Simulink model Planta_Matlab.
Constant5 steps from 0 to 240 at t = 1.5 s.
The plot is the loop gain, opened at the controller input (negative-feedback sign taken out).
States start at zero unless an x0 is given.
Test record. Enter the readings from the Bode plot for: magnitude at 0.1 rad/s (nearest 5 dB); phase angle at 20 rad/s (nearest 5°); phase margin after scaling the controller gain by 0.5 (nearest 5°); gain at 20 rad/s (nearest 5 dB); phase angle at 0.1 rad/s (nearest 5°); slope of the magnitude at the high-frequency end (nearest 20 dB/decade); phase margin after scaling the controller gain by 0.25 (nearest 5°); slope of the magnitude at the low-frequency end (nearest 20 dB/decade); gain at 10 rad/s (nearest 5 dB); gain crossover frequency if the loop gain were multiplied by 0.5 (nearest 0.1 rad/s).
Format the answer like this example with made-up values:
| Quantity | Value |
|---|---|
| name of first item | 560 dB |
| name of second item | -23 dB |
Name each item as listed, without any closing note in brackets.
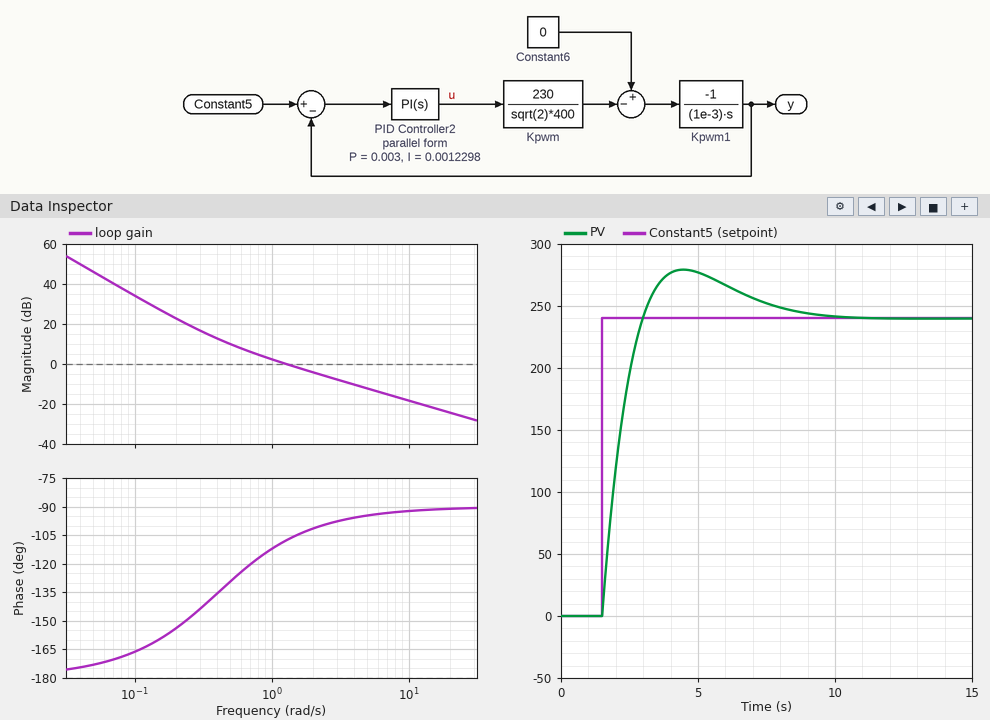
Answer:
| Quantity | Value |
|---|---|
| magnitude at 0.1 rad/s | 35 dB |
| phase angle at 20 rad/s | -90° |
| phase margin after scaling the controller gain by 0.5 | 60° |
| gain at 20 rad/s | -25 dB |
| phase angle at 0.1 rad/s | -165° |
| slope of the magnitude at the high-frequency end | -20 dB/decade |
| phase margin after scaling the controller gain by 0.25 | 45° |
| slope of the magnitude at the low-frequency end | -40 dB/decade |
| gain at 10 rad/s | -20 dB |
| gain crossover frequency if the loop gain were multiplied by 0.5 | 0.7 rad/s |
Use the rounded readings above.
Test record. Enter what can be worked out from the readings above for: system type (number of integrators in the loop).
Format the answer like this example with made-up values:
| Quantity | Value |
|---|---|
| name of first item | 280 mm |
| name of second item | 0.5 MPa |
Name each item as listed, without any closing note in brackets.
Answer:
| Quantity | Value |
|---|---|
| system type | 2 |
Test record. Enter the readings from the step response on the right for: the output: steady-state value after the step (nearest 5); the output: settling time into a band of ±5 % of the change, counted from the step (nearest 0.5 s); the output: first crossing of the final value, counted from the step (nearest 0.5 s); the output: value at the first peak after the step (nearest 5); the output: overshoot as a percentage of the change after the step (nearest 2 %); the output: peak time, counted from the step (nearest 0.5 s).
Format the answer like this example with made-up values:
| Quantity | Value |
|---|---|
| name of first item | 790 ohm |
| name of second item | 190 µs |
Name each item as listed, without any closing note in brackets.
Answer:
| Quantity | Value |
|---|---|
| the output: steady-state value after the step | 240 |
| the output: settling time into a band of ±5 % of the change, counted from the step | 6.0 s |
| the output: first crossing of the final value, counted from the step | 1.5 s |
| the output: value at the first peak after the step | 280 |
| the output: overshoot as a percentage of the change after the step | 16 % |
| the output: peak time, counted from the step | 3.0 s |
